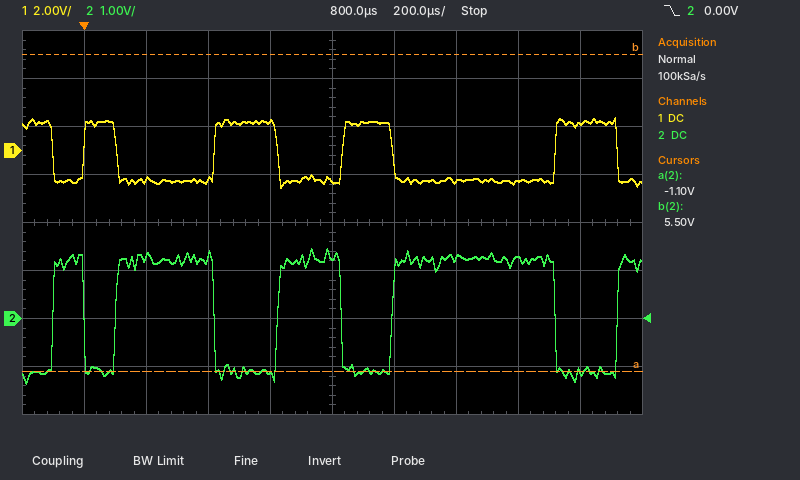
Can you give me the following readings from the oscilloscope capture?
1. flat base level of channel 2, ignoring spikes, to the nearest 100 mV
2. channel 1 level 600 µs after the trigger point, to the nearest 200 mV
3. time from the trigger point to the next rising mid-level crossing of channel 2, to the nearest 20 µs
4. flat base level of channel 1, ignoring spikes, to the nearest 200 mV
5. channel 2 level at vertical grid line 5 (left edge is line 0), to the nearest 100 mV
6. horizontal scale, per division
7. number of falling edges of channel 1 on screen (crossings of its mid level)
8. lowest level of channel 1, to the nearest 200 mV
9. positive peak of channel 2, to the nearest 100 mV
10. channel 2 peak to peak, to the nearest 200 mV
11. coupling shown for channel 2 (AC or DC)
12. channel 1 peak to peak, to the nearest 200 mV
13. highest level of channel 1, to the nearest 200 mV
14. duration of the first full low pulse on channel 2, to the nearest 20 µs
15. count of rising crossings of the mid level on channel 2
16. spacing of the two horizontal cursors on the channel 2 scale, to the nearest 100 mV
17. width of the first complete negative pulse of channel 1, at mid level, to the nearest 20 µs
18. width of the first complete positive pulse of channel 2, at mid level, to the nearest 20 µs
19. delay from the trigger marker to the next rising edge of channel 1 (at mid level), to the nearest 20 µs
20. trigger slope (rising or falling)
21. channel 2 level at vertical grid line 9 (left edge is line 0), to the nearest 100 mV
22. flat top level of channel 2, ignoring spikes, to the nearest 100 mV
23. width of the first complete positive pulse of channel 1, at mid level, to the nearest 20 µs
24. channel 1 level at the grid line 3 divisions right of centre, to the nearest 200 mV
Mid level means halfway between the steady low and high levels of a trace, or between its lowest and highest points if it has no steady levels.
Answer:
-1.1 V
1.2 V
100 µs
-1.2 V
1.3 V
200 µs
5
-1.6 V
1.5 V
2.8 V
DC
3.0 V
1.4 V
100 µs
5
6.6 V
100 µs
100 µs
420 µs
falling
-1.1 V
1.2 V
100 µs
-1.2 V
